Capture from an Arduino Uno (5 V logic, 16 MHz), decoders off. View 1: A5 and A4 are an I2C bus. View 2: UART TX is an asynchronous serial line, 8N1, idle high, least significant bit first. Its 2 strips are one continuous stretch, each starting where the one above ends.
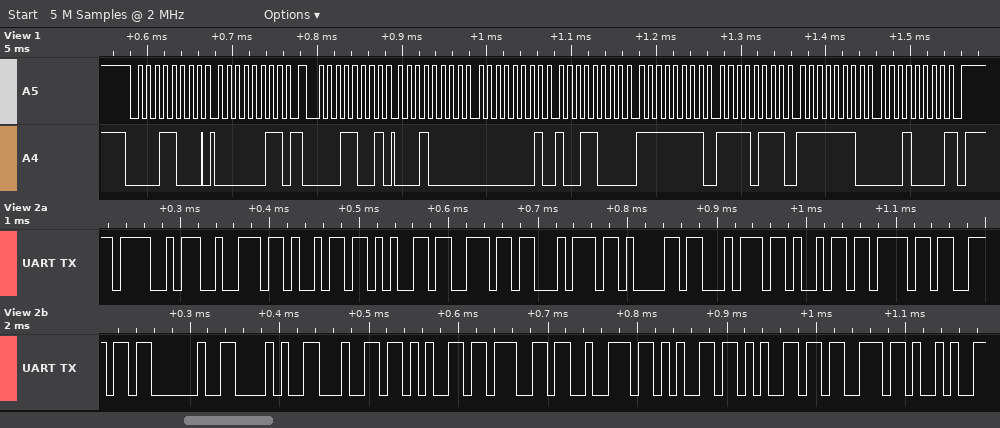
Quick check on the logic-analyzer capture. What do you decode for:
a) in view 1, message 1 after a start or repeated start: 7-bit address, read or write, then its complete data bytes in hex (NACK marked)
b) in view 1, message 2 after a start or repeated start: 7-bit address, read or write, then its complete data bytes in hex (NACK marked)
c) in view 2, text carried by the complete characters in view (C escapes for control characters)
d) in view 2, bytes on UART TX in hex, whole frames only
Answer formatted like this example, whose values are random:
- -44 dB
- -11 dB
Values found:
- 0x0C write: 03
- 0x0C read: 10 01 98 FF F7 FE 10 NACK
- "Orientation (degrees)"
- 4F 72 69 65 6E 74 61 74 69 6F 6E 20 28 64 65 67 72 65 65 73 29
